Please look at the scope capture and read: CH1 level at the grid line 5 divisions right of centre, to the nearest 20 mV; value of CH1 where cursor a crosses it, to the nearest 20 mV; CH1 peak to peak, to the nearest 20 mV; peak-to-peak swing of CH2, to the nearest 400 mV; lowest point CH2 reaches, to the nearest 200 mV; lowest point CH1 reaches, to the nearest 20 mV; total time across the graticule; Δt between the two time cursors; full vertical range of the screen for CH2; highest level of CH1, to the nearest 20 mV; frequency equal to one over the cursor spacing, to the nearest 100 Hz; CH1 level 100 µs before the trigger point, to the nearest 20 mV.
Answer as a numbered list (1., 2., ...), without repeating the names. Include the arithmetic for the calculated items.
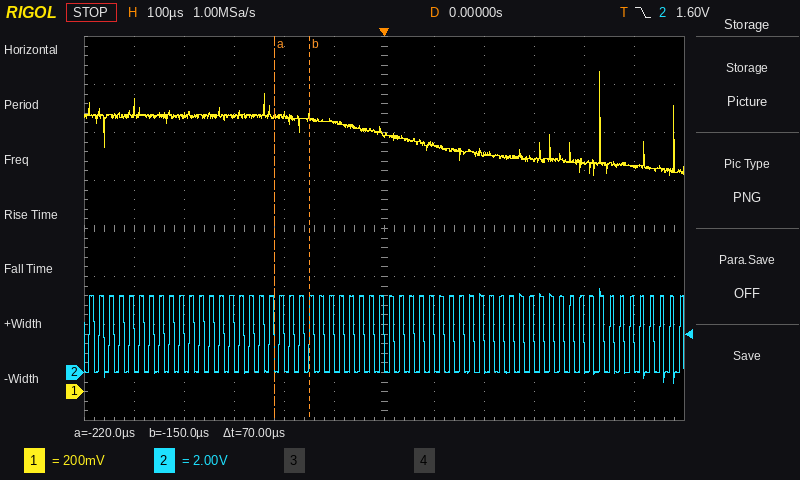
1. 940 mV
2. 1.14 V
3. 1.34 V − (900 mV) = 440 mV
4. 4.0 V
5. -400 mV
6. 900 mV
7. 1.2 ms
8. 70 µs
9. 16 V
10. 1.34 V
11. 1 / 70 µs ≈ 14.3 kHz
12. 1.12 V
